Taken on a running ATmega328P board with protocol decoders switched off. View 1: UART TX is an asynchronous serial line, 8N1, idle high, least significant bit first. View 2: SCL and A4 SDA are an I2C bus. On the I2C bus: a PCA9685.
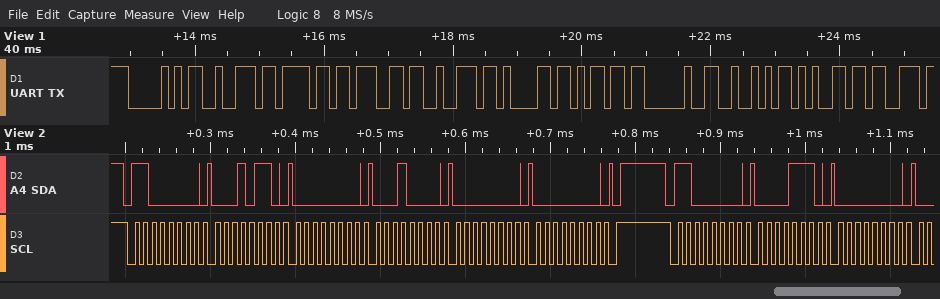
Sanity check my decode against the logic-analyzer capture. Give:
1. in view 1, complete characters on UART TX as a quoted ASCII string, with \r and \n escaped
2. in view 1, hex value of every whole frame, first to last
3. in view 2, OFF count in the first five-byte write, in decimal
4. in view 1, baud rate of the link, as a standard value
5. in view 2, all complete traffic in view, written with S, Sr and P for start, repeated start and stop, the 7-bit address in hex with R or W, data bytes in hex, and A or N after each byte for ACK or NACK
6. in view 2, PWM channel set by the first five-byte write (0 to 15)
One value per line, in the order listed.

"Program Res"
0x50 0x72 0x6F 0x67 0x72 0x61 0x6D 0x20 0x52 0x65 0x73
0
9600 baud
S 60W A 16 A 00 A 10 A 00 A 00 A P S 60W A 0E A 00 A
4
